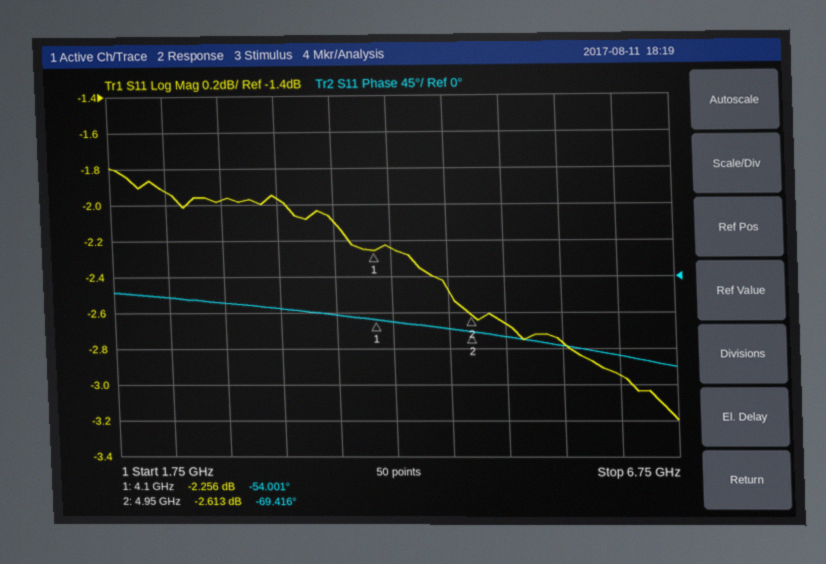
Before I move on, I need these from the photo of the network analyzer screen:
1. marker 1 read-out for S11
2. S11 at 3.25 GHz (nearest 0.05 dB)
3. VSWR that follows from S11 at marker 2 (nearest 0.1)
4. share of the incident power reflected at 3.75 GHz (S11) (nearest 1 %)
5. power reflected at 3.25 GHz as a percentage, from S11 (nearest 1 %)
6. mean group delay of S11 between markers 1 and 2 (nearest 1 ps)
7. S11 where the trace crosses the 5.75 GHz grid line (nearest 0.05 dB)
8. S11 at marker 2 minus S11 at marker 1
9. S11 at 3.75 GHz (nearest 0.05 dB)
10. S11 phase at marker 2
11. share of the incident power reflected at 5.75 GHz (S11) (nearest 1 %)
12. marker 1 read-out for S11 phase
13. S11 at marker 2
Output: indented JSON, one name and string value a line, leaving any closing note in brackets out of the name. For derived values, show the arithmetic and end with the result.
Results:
{
  "marker 1 read-out for S11": "-2.256 dB",
  "S11 at 3.25 GHz": "-1.95 dB",
  "VSWR that follows from S11 at marker 2": "(1 + 0.7402)/(1 − 0.7402) ≈ 6.7",
  "share of the incident power reflected at 3.75 GHz (S11)": "10^(-2.1/10) ≈ 62 %",
  "power reflected at 3.25 GHz as a percentage, from S11": "10^(-1.95/10) ≈ 64 %",
  "mean group delay of S11 between markers 1 and 2": "−(-69.416° − (-54.001°))/(360° × 850 MHz) ≈ 50 ps",
  "S11 where the trace crosses the 5.75 GHz grid line": "-2.75 dB",
  "S11 at marker 2 minus S11 at marker 1": "-2.613 − (-2.256) = -0.357 dB",
  "S11 at 3.75 GHz": "-2.10 dB",
  "S11 phase at marker 2": "-69.416°",
  "share of the incident power reflected at 5.75 GHz (S11)": "10^(-2.75/10) ≈ 53 %",
  "marker 1 read-out for S11 phase": "-54.001°",
  "S11 at marker 2": "-2.613 dB"
}
